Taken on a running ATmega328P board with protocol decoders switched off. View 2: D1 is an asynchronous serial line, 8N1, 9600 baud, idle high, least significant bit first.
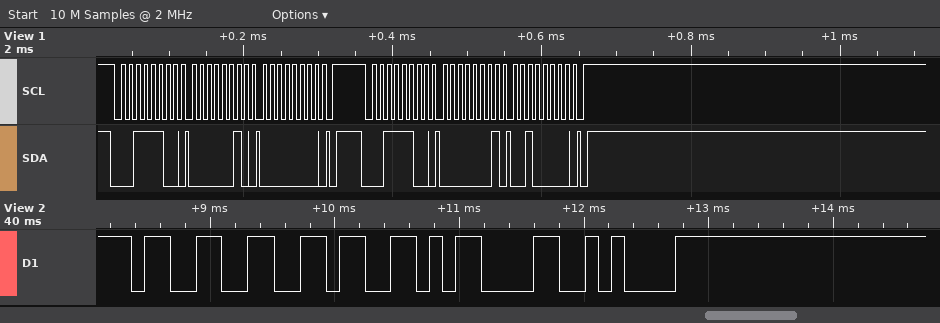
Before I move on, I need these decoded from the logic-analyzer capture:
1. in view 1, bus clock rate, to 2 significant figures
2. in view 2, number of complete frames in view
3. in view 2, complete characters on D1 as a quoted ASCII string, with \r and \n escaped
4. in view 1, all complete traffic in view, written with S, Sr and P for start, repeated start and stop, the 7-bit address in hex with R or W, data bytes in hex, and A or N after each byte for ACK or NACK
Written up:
100 kHz
4
"36\r\n"
S 1EW A 02 A 00 A P S 1EW A 01 A 20 A P
